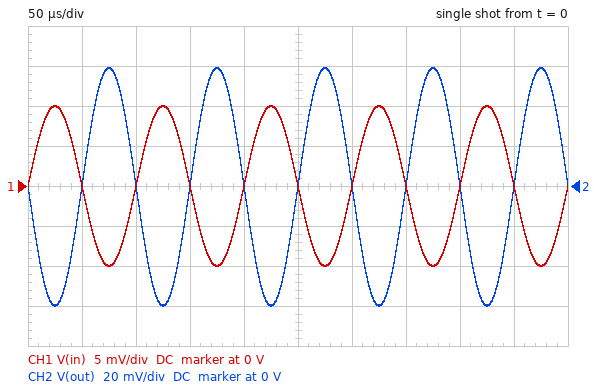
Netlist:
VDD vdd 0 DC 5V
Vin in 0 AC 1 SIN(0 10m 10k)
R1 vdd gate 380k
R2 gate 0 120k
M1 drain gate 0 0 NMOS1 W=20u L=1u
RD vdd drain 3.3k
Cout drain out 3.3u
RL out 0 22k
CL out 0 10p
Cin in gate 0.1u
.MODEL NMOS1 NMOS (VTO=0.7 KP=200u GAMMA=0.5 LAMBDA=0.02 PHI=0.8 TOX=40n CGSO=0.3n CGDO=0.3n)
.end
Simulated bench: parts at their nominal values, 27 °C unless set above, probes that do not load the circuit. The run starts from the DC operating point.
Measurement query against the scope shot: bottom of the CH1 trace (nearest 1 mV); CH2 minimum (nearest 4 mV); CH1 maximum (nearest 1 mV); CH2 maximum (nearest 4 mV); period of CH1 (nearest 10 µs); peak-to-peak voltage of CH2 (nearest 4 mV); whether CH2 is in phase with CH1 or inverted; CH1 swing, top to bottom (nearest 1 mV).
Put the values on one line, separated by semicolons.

-10 mV; -60 mV; 10 mV; 60 mV; 100 µs; 120 mV; inverted; 20 mV
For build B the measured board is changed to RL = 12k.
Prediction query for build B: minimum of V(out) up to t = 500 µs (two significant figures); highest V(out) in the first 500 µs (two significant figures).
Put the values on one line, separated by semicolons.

-54 mV; 53 mV
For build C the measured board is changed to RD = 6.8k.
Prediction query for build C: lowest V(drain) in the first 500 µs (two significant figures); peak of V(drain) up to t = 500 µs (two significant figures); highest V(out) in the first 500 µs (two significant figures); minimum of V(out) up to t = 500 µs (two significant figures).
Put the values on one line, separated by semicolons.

1.4 V; 1.6 V; 100 mV; -100 mV
